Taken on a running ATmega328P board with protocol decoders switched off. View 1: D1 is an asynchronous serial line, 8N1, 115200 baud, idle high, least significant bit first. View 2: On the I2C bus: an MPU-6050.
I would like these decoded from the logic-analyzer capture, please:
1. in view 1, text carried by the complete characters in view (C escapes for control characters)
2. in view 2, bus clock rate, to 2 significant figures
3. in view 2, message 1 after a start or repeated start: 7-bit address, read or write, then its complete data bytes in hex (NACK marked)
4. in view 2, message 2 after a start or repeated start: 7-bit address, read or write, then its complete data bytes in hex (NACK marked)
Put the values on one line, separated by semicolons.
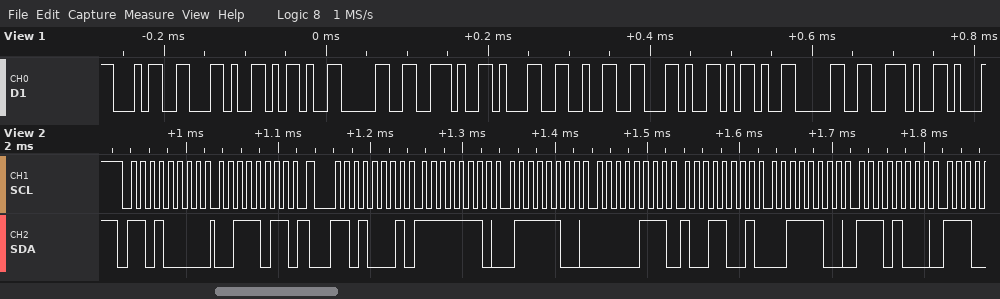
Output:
"4,-0.12,-0."; 100 kHz; 0x68 write: 3B; 0x68 read: FE 7C 07 99 3C E8
